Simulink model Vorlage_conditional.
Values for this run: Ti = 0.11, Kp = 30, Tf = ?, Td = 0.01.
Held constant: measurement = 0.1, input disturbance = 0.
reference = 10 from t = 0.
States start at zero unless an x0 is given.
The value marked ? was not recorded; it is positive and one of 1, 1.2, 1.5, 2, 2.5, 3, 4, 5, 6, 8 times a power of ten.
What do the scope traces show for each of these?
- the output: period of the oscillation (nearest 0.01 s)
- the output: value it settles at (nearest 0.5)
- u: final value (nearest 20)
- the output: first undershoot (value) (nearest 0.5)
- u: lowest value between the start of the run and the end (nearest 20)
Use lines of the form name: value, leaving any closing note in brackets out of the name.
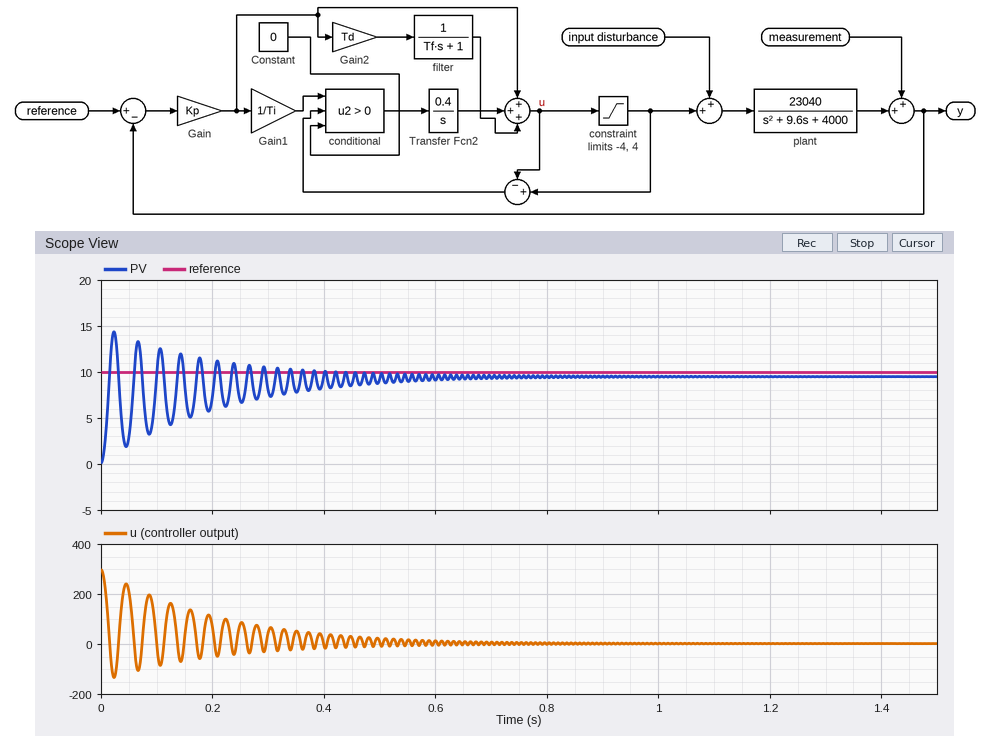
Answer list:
the output: period of the oscillation: 0.04 s
the output: value it settles at: 9.5
u: final value: 0
the output: first undershoot (value): 2.0
u: lowest value between the start of the run and the end: -140
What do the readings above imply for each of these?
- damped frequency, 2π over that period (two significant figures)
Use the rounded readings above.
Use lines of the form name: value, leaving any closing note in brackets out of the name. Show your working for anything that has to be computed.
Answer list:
damped frequency, 2π over that period: 2π / 0.04 = 160 rad/s
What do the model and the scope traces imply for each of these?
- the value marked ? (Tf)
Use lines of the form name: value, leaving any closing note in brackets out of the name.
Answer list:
the value marked ?: 0.005
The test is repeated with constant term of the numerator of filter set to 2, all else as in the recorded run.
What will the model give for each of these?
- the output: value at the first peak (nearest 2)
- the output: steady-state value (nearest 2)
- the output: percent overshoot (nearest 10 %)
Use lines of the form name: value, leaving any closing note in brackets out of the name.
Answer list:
the output: value at the first peak: 14
the output: steady-state value: 10
the output: percent overshoot: 50 %
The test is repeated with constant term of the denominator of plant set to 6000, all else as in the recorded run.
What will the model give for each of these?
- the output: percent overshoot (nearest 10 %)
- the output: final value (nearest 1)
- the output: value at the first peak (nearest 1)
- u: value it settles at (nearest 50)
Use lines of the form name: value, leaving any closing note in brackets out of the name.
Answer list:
the output: percent overshoot: 40 %
the output: final value: 10
the output: value at the first peak: 13
u: value it settles at: 0
